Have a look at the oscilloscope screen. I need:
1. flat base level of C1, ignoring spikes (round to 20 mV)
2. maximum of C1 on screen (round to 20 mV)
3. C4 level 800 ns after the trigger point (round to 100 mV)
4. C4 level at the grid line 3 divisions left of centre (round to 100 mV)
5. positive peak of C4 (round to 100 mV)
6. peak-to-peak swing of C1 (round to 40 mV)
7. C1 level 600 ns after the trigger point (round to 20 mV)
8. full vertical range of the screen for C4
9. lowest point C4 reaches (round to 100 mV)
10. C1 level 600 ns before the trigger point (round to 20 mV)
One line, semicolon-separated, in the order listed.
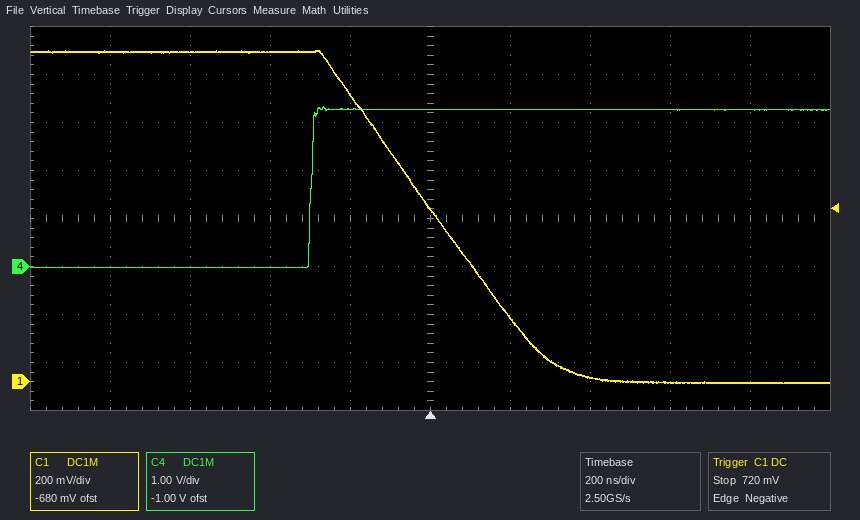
0 mV; 1.38 V; 3.3 V; 0.0 V; 3.3 V; 1.40 V; 0 mV; 8 V; 0.0 V; 1.38 V
